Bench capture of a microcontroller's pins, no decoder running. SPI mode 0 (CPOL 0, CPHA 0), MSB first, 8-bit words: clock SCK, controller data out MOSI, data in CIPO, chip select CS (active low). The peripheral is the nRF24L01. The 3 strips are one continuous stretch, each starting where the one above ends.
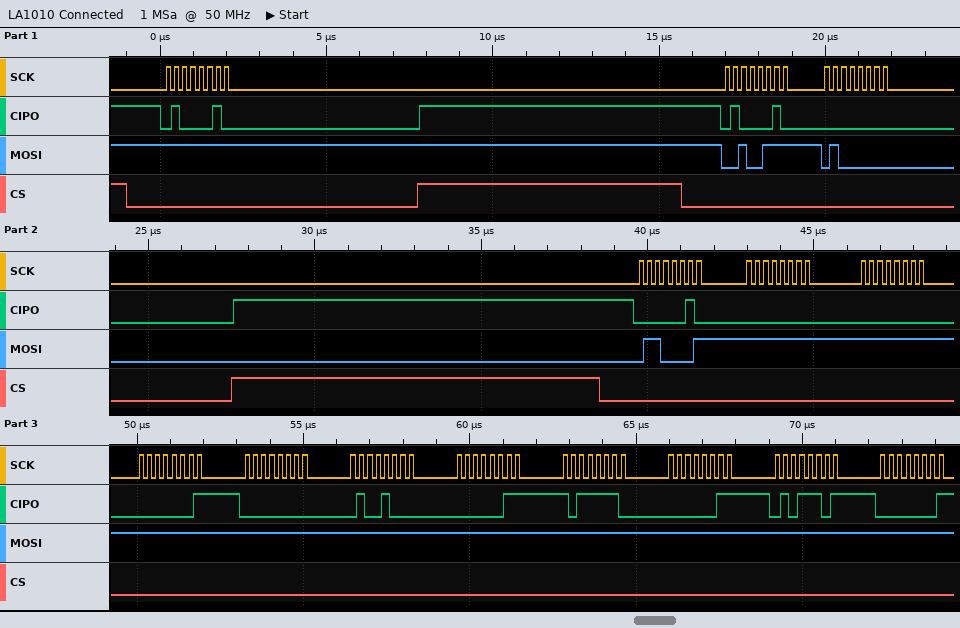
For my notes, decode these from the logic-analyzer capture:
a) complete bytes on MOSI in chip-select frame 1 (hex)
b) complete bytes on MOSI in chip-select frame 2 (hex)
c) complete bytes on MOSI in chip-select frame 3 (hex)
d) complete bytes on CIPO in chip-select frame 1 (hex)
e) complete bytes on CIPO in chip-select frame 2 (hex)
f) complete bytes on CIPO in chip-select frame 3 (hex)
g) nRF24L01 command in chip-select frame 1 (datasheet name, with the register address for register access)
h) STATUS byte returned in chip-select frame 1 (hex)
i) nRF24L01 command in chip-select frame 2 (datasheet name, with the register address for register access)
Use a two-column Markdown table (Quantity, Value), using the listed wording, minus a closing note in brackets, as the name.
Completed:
| Quantity | Value |
|---|---|
| complete bytes on MOSI in chip-select frame 1 | 0xFF |
| complete bytes on MOSI in chip-select frame 2 | 0x27 0x40 |
| complete bytes on MOSI in chip-select frame 3 | 0x61 0xFF 0xFF 0xFF 0xFF 0xFF 0xFF 0xFF 0xFF 0xFF 0xFF |
| complete bytes on CIPO in chip-select frame 1 | 0x42 |
| complete bytes on CIPO in chip-select frame 2 | 0x42 0x00 |
| complete bytes on CIPO in chip-select frame 3 | 0x02 0x00 0x00 0x01 0x00 0x48 0x03 0xBE 0x03 0x5D 0x01 |
| nRF24L01 command in chip-select frame 1 | NOP |
| STATUS byte returned in chip-select frame 1 | 0x42 |
| nRF24L01 command in chip-select frame 2 | W_REGISTER 0x07 |
